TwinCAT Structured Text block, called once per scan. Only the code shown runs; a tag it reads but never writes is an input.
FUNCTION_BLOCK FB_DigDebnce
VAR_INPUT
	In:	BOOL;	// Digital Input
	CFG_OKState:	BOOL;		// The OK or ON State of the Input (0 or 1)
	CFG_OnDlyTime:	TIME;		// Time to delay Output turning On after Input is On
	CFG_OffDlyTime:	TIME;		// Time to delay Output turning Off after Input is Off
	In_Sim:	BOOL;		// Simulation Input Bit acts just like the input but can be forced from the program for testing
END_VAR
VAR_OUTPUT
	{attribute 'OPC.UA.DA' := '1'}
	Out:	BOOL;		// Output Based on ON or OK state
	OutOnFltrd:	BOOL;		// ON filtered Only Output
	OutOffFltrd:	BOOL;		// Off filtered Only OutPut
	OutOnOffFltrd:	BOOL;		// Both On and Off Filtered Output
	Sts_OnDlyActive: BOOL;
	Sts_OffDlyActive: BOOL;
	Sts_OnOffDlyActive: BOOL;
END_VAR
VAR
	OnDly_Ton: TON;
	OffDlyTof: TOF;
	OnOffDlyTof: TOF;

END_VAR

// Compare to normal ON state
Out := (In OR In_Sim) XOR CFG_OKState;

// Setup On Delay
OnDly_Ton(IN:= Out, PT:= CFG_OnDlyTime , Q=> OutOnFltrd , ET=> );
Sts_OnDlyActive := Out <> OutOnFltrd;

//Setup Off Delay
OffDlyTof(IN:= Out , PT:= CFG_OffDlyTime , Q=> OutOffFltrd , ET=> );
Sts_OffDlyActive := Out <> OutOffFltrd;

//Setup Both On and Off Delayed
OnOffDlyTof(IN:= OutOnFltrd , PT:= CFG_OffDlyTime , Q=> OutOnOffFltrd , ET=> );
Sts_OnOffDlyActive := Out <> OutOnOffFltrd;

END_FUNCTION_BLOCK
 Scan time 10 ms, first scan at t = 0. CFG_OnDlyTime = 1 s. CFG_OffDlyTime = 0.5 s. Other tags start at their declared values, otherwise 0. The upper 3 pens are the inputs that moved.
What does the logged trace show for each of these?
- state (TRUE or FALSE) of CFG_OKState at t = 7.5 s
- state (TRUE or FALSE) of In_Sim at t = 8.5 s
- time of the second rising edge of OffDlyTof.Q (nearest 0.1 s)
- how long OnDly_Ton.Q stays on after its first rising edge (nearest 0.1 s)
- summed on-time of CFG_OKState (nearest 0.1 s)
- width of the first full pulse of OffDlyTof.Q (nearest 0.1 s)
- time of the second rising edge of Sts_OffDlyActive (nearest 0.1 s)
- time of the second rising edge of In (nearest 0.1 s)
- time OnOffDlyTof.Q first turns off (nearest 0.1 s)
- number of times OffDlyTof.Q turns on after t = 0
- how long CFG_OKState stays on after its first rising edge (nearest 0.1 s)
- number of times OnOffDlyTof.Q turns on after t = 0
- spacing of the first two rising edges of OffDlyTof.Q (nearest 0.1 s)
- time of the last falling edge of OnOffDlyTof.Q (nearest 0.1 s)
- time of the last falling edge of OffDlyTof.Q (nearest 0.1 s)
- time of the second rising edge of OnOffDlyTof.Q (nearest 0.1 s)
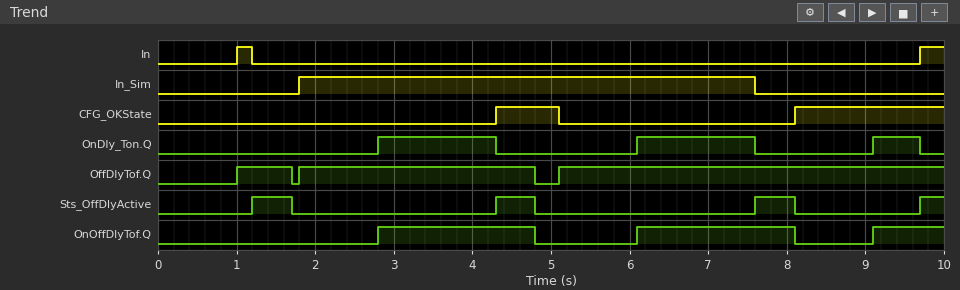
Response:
FALSE
FALSE
1.8 s
1.5 s
2.7 s
0.7 s
4.3 s
9.7 s
4.8 s
3
0.8 s
3
0.8 s
8.1 s
4.8 s
6.1 s
